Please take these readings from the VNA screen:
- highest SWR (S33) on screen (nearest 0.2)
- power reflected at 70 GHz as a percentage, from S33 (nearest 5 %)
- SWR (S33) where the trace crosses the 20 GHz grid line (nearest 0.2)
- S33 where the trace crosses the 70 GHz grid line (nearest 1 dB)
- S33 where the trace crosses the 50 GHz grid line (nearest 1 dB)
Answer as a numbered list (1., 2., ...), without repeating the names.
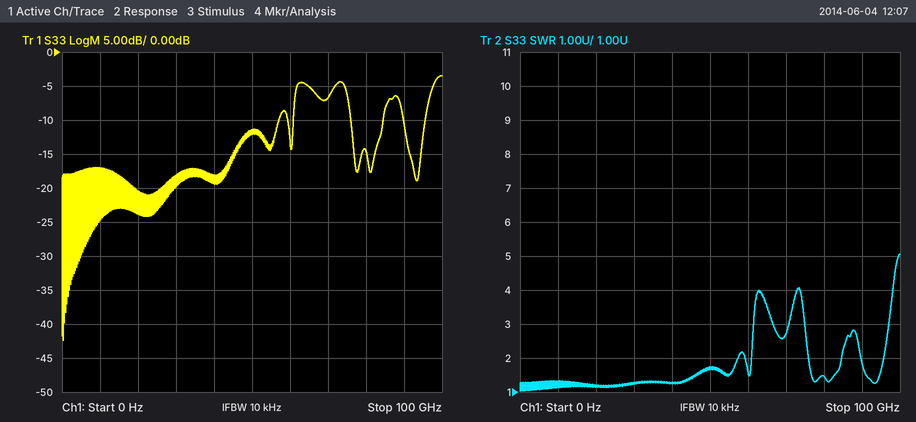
1. 5.0
2. 20 %
3. 1.2
4. -7 dB
5. -12 dB
